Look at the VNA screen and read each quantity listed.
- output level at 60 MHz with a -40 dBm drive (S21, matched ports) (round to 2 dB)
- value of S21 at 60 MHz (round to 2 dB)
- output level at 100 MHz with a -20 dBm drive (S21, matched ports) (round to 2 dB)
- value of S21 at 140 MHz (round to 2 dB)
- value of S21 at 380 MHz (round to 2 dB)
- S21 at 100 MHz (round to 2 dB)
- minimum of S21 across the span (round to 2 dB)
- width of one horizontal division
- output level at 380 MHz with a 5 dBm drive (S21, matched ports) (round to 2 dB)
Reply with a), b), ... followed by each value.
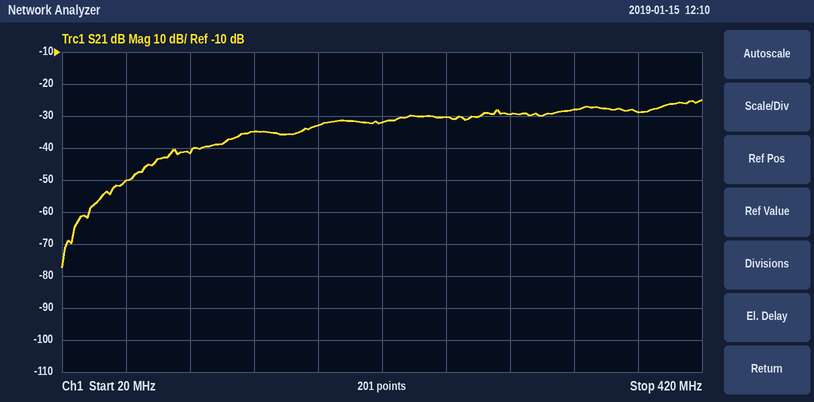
a) -90 dBm
b) -50 dB
c) -62 dBm
d) -34 dB
e) -28 dB
f) -42 dB
g) -78 dB
h) 40 MHz
i) -24 dBm
